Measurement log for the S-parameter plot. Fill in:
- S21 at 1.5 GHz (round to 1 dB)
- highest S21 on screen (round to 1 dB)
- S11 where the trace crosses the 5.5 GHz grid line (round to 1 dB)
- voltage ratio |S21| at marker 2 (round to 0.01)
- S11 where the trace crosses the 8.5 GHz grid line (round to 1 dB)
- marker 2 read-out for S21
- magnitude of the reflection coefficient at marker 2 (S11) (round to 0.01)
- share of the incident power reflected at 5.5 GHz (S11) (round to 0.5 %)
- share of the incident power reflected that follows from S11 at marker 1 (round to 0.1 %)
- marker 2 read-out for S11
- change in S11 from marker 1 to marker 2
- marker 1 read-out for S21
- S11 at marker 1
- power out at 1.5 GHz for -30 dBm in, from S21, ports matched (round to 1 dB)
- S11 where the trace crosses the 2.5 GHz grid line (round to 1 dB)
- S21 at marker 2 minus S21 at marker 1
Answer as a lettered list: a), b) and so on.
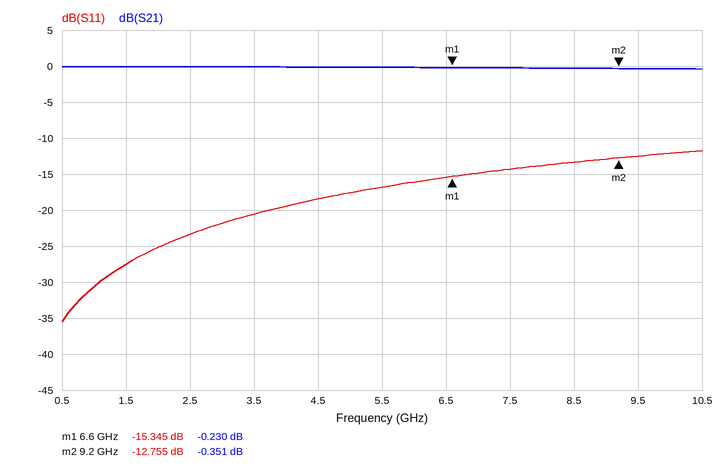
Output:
a) 0 dB
b) 0 dB
c) -17 dB
d) 0.96
e) -13 dB
f) -0.351 dB
g) 0.23
h) 2.0 %
i) 2.9 %
j) -12.755 dB
k) 2.590 dB
l) -0.230 dB
m) -15.345 dB
n) -30 dBm
o) -23 dB
p) -0.121 dB
